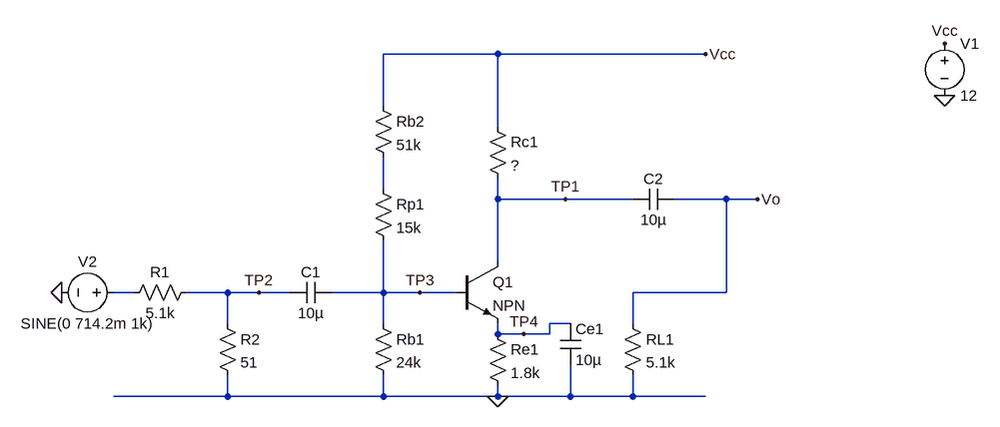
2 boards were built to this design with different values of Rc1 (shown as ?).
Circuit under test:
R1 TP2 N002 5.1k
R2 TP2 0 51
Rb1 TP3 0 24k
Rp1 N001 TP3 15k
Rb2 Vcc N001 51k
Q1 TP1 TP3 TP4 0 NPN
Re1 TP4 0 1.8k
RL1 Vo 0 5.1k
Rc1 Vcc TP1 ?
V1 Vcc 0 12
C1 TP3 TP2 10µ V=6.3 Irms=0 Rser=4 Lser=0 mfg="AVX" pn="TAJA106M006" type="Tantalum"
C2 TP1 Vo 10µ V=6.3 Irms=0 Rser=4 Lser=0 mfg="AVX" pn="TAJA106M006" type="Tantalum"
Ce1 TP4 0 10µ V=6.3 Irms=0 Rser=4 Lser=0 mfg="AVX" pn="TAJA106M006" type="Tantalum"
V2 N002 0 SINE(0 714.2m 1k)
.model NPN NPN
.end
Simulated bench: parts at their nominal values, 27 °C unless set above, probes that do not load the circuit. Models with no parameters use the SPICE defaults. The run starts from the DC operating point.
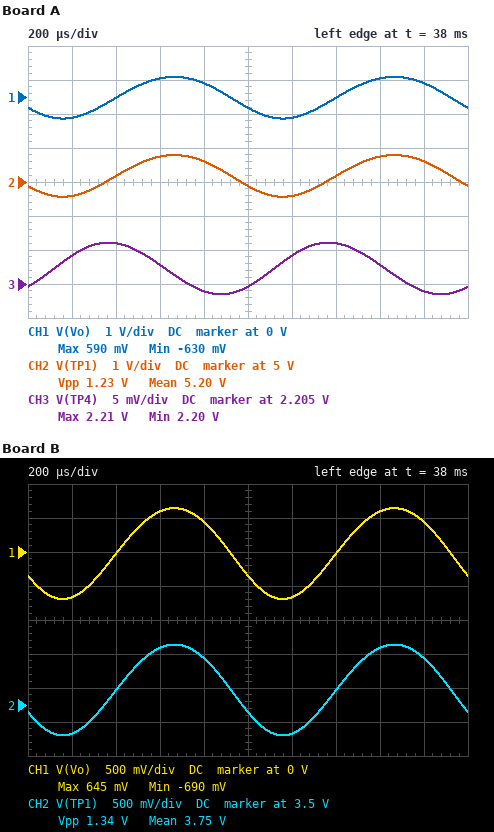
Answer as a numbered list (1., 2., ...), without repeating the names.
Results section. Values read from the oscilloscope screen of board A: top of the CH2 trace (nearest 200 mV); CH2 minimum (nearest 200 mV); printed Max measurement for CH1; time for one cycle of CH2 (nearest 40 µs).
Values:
1. 5.8 V
2. 4.6 V
3. 590 mV
4. 1.00 ms
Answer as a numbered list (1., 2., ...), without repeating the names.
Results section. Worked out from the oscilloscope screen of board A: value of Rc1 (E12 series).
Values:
1. 5.6 kΩ
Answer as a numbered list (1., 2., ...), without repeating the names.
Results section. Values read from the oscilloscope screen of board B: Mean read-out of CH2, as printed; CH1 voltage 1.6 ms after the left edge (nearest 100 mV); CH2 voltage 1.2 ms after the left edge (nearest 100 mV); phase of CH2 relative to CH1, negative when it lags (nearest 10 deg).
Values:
1. 3.75 V
2. 600 mV
3. 3.1 V
4. 0 deg
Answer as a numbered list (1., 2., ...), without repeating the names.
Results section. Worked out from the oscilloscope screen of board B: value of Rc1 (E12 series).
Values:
1. 6.8 kΩ
